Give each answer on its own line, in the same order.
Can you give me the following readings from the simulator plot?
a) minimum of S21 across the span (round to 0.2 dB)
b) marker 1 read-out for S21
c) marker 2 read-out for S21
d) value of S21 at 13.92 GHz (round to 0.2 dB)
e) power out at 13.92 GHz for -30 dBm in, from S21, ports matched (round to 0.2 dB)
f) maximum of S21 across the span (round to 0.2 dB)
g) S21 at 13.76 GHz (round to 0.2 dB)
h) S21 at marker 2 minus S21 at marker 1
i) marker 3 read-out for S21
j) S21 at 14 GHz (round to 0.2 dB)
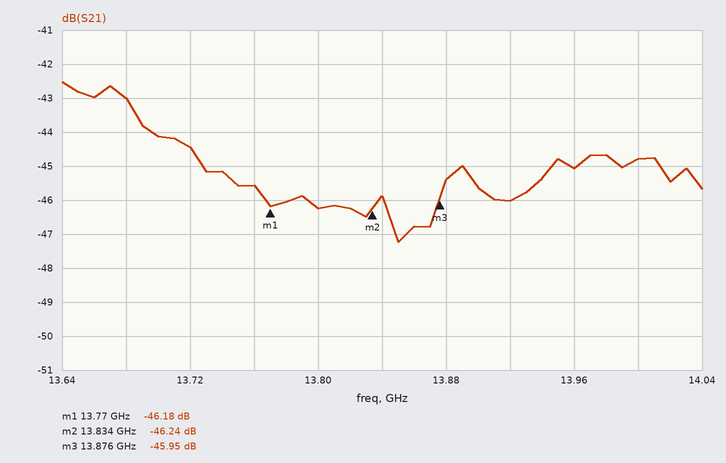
-47.2 dB
-46.18 dB
-46.24 dB
-46.0 dB
-76.0 dBm
-42.6 dB
-45.6 dB
-0.06 dB
-45.95 dB
-44.8 dB
